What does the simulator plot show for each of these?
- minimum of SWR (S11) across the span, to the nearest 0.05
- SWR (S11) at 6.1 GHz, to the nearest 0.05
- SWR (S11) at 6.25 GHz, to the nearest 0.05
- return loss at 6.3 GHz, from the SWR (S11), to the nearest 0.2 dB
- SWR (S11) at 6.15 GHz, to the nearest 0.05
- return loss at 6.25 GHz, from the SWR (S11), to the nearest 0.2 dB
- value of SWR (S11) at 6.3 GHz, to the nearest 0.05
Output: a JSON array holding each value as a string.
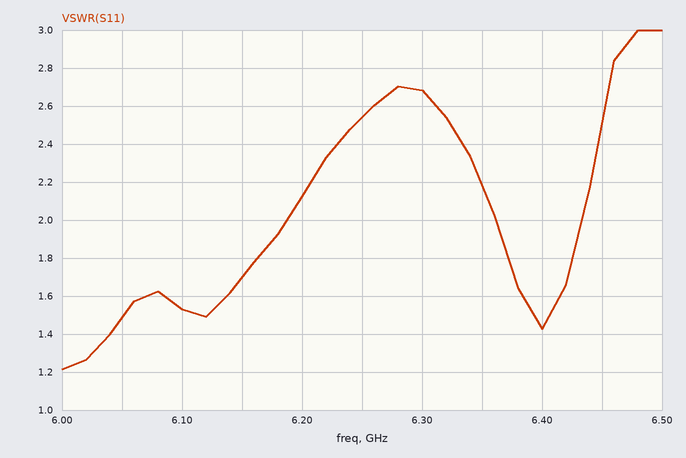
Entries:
["1.20", "1.55", "2.55", "6.8 dB", "1.70", "7.2 dB", "2.70"]
